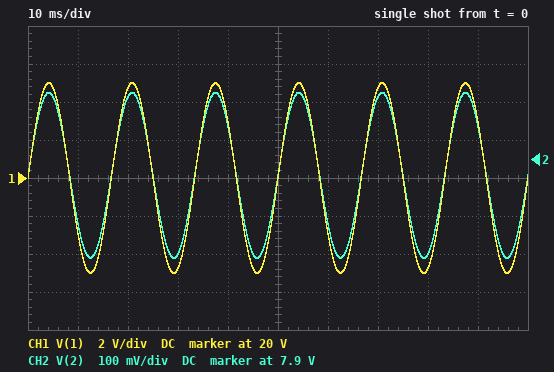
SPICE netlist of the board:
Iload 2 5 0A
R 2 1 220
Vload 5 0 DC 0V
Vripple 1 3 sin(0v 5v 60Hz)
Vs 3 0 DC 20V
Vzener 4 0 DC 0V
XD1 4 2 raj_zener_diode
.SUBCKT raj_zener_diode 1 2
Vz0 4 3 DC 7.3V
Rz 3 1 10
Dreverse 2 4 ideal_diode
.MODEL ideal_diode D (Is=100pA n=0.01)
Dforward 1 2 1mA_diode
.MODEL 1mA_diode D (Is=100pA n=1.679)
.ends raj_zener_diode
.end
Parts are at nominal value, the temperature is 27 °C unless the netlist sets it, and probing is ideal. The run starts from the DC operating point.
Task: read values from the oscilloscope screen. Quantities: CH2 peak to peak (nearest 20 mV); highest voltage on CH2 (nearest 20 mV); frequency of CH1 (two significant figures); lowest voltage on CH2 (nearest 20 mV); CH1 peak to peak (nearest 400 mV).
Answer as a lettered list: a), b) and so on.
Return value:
a) 440 mV
b) 8.08 V
c) 60 Hz
d) 7.64 V
e) 10.0 V
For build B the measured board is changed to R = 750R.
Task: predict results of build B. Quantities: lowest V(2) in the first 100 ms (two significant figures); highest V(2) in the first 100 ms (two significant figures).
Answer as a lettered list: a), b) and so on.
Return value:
a) 7.4 V
b) 7.5 V
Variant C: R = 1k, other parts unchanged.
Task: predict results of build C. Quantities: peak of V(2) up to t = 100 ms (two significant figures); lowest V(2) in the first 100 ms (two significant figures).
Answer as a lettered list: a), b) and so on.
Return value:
a) 7.5 V
b) 7.4 V
